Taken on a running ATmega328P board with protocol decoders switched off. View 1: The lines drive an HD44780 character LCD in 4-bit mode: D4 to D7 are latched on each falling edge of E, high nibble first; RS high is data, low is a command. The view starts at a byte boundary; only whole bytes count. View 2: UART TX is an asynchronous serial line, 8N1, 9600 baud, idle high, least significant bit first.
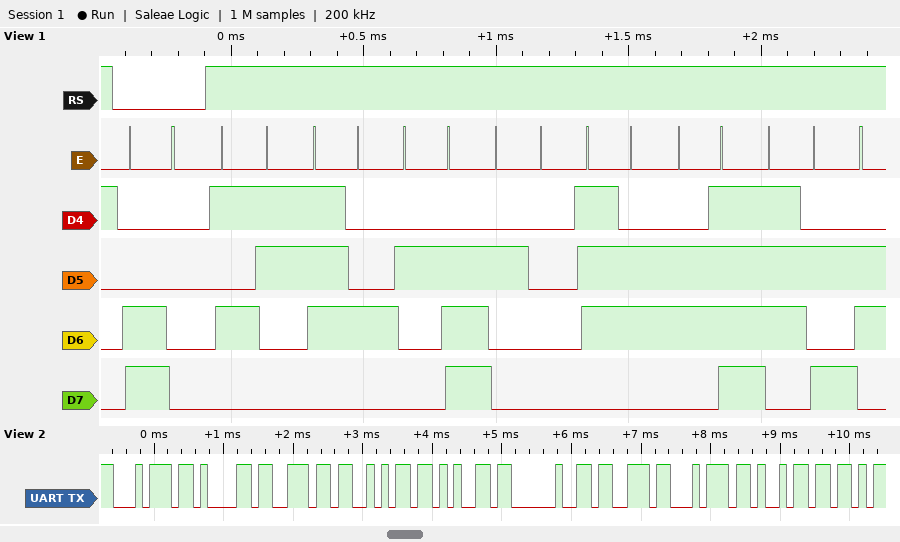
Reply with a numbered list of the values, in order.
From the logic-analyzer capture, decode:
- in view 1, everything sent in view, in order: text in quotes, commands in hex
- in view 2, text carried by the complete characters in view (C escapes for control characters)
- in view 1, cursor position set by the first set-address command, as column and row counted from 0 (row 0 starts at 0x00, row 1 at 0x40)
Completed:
1. 0xC0 "St. voz"
2. "tanje sti"
3. column 0, row 1
